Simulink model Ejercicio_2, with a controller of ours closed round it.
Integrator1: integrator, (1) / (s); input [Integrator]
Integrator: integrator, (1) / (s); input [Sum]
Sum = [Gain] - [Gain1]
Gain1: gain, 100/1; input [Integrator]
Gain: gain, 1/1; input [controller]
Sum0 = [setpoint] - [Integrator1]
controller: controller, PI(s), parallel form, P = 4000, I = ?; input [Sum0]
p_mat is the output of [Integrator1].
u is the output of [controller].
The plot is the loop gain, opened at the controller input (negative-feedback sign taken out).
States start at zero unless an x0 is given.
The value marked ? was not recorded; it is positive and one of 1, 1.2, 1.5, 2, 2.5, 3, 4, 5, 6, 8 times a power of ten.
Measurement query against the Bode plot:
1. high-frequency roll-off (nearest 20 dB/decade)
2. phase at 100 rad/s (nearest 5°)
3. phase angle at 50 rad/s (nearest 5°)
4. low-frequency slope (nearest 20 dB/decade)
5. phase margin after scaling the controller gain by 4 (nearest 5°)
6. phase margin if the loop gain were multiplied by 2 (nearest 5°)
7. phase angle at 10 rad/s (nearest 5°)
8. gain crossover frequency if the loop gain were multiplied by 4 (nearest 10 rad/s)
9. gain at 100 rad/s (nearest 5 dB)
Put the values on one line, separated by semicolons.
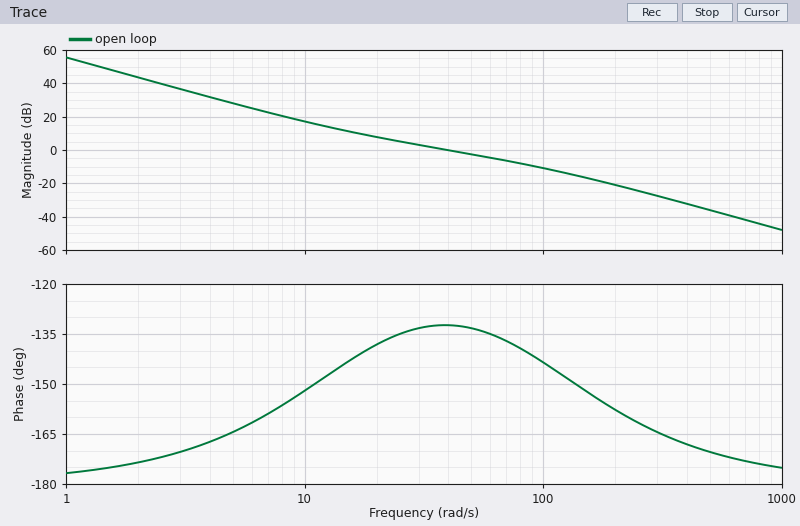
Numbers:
-40 dB/decade; -145°; -135°; -40 dB/decade; 35°; 45°; -150°; 110 rad/s; -10 dB
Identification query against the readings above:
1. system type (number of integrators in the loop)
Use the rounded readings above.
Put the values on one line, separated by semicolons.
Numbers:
2
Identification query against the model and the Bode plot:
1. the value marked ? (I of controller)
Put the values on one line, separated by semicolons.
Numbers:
60000
